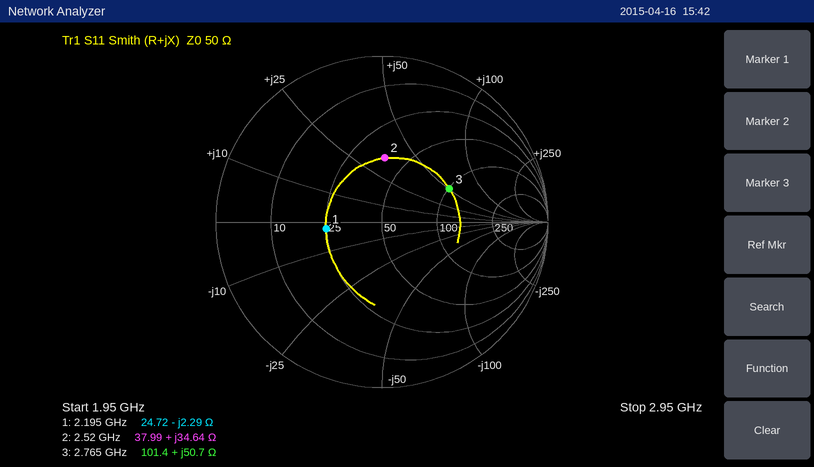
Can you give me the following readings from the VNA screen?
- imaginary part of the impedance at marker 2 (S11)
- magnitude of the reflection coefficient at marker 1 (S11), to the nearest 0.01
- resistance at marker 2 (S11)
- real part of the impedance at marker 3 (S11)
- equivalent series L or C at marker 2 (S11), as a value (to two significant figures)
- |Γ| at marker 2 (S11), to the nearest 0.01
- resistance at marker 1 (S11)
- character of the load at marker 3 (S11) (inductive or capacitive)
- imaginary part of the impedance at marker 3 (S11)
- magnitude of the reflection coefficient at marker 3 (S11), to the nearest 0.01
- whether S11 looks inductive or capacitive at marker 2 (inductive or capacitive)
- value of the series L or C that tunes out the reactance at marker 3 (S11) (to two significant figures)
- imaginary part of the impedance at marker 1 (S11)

+34.64 Ω
0.34
37.99 Ω
101.4 Ω
2.2 nH
0.39
24.72 Ω
inductive
+50.7 Ω
0.45
inductive
1.1 pF
-2.29 Ω
